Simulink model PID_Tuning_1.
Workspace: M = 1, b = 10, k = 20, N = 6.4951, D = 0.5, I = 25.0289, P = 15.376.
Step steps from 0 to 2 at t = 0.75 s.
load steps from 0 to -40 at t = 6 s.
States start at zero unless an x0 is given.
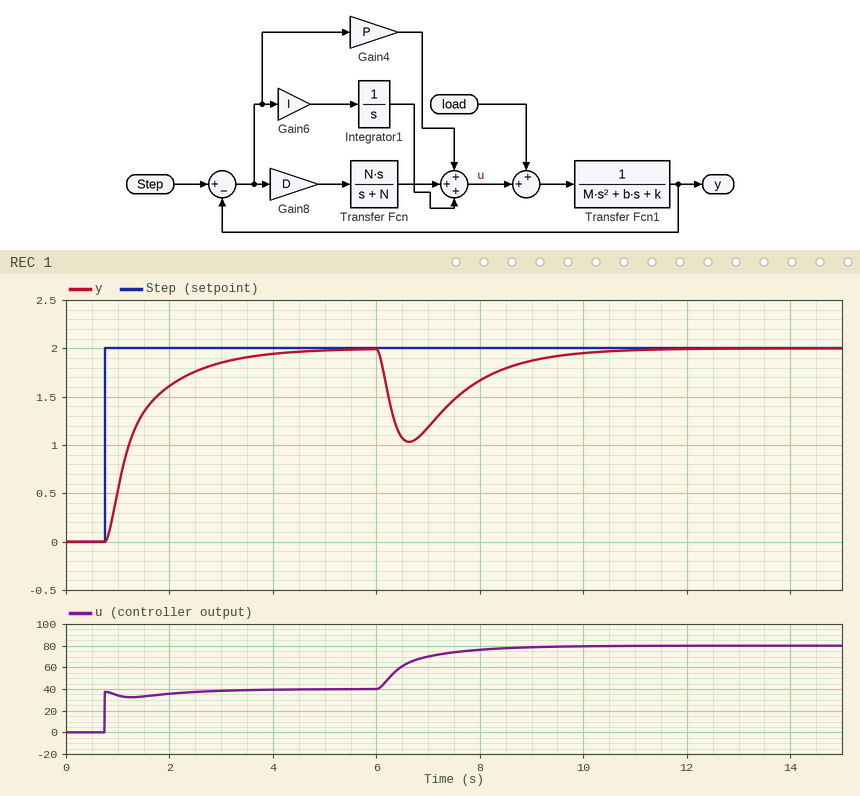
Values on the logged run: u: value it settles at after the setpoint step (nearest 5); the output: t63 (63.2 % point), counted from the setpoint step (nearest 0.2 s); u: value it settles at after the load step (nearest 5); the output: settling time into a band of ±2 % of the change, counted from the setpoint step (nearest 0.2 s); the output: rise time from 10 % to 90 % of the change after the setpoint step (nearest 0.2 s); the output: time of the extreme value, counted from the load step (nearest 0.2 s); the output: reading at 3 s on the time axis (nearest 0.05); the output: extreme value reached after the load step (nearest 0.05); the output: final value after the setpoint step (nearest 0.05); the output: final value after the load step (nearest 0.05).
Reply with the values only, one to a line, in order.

40
0.6 s
80
3.6 s
1.8 s
0.6 s
1.85
1.05
2.00
2.00
